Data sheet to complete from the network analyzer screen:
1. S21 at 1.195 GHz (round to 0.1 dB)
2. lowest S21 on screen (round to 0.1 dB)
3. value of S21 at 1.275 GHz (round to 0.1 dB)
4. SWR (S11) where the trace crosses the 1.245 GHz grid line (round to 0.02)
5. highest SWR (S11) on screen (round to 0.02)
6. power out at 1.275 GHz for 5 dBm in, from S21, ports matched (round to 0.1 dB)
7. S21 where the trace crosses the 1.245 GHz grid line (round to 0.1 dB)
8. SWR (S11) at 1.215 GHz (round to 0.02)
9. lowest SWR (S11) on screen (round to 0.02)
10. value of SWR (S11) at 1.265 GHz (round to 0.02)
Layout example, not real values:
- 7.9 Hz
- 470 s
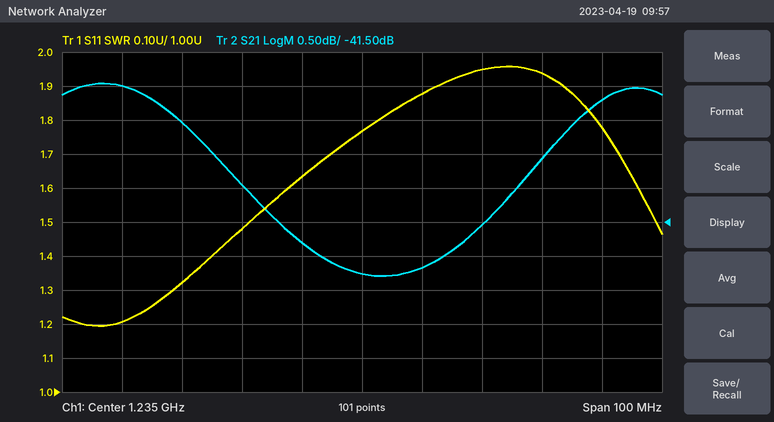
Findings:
- -39.5 dB
- -42.3 dB
- -39.7 dB
- 1.88
- 1.96
- -34.7 dBm
- -42.2 dB
- 1.48
- 1.20
- 1.94
